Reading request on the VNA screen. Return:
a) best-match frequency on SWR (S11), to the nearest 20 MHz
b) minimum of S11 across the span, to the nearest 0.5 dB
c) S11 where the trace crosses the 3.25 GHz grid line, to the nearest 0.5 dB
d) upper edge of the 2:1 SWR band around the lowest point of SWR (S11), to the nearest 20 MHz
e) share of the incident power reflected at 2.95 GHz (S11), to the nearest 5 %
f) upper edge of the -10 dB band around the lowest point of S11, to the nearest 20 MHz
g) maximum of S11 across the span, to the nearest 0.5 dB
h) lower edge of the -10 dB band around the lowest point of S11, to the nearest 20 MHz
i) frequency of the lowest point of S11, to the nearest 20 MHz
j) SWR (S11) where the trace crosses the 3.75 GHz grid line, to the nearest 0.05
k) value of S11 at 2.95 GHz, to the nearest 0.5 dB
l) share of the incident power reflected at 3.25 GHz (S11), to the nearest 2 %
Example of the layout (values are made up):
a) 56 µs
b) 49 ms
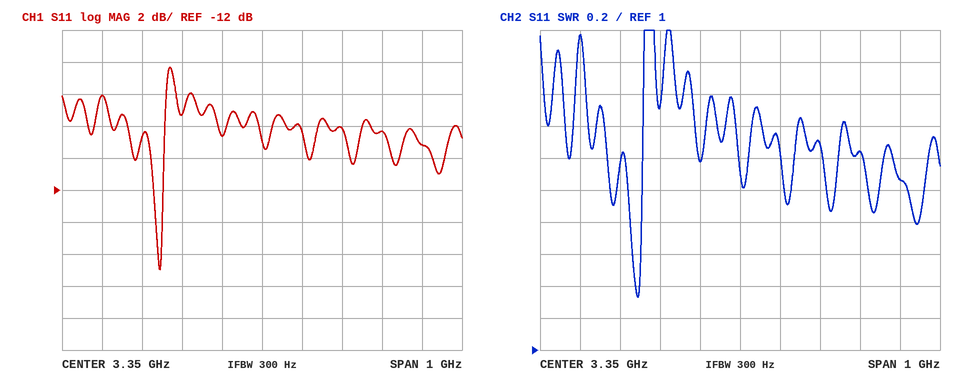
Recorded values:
a) 3.10 GHz
b) -17.0 dB
c) -8.5 dB
d) 3.10 GHz
e) 25 %
f) 3.10 GHz
g) -4.5 dB
h) 3.08 GHz
i) 3.10 GHz
j) 2.05
k) -6.0 dB
l) 14 %
